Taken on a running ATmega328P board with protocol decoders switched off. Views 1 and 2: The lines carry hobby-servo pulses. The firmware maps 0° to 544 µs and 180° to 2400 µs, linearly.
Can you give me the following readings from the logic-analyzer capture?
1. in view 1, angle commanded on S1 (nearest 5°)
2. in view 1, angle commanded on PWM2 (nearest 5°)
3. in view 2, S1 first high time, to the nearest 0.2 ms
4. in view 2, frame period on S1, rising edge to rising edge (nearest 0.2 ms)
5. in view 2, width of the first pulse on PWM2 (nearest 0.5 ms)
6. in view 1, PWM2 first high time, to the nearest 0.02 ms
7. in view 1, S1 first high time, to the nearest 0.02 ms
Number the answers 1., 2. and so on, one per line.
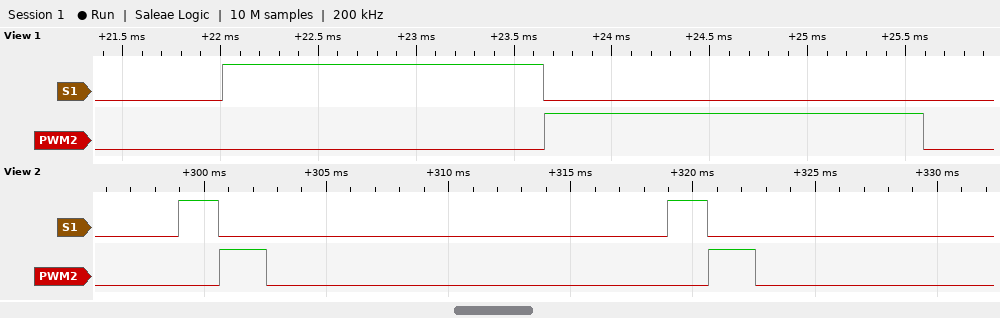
1. 105°
2. 135°
3. 1.6 ms
4. 20.0 ms
5. 2.0 ms
6. 1.94 ms
7. 1.64 ms
